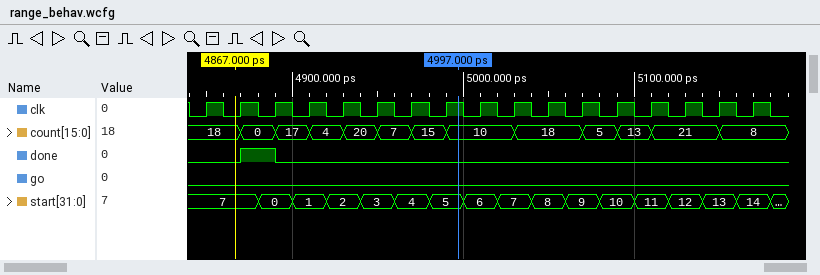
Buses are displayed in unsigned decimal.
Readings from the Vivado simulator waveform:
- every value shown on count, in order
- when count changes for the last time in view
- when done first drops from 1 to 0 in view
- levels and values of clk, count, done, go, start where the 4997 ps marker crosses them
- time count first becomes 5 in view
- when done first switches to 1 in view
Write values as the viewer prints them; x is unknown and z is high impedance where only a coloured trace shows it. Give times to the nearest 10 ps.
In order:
18, 0, 17, 4, 20, 7, 15, 10, 18, 5, 13, 21, 8
5150 ps
4890 ps
clk=1, count=10, done=0, go=0, start=5
5070 ps
4870 ps
